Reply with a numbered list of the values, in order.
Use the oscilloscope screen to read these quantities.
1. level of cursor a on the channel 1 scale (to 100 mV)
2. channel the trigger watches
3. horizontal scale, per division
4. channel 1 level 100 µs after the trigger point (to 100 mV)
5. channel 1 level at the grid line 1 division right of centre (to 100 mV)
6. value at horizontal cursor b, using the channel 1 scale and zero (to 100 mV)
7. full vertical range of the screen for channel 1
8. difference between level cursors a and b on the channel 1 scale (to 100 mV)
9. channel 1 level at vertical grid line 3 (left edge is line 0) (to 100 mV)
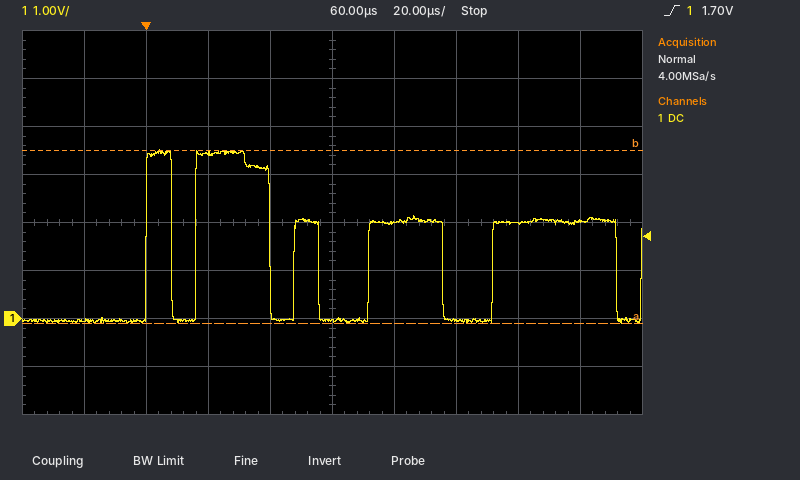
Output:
1. -100 mV
2. channel 1
3. 20 µs
4. 0.0 V
5. 2.0 V
6. 3.5 V
7. 8 V
8. 3.6 V
9. 3.4 V
